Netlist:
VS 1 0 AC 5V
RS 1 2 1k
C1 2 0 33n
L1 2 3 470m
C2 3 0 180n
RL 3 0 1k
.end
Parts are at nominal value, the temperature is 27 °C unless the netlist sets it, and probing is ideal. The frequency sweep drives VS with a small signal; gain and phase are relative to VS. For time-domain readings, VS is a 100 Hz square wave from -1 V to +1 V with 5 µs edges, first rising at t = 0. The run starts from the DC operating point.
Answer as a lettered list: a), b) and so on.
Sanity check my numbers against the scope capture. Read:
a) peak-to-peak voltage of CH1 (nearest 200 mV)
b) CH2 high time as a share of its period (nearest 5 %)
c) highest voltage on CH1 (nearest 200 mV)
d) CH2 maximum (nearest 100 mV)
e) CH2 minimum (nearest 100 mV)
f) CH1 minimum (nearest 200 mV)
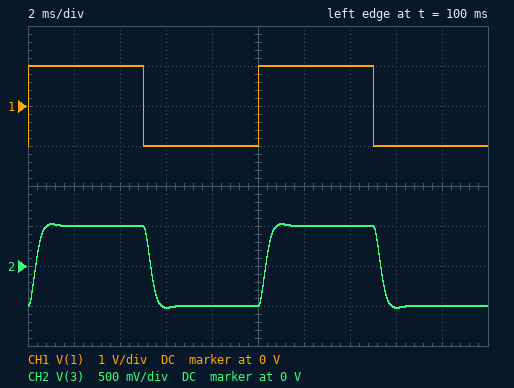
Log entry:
a) 2.0 V
b) 50 %
c) 1.0 V
d) 500 mV
e) -500 mV
f) -1.0 V
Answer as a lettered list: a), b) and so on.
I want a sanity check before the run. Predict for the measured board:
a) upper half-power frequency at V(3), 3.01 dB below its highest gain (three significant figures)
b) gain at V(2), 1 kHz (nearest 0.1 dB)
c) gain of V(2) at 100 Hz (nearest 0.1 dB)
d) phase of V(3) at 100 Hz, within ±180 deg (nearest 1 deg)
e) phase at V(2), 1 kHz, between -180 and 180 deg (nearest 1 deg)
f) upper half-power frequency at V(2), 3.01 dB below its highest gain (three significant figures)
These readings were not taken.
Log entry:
a) 719 Hz
b) -0.7 dB
c) -6.0 dB
d) -12 deg
e) 10 deg
f) 5.30 kHz
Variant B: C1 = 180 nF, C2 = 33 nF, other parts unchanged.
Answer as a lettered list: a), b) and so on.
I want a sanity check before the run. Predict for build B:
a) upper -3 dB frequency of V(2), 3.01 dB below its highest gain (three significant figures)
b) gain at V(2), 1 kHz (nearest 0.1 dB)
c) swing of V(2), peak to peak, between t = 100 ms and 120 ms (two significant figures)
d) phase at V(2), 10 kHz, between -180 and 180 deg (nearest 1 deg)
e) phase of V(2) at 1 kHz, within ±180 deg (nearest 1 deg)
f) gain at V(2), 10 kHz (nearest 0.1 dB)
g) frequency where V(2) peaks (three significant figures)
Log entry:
a) 1.49 kHz
b) -2.8 dB
c) 1.8 V
d) -85 deg
e) -36 deg
f) -21.1 dB
g) 707 Hz
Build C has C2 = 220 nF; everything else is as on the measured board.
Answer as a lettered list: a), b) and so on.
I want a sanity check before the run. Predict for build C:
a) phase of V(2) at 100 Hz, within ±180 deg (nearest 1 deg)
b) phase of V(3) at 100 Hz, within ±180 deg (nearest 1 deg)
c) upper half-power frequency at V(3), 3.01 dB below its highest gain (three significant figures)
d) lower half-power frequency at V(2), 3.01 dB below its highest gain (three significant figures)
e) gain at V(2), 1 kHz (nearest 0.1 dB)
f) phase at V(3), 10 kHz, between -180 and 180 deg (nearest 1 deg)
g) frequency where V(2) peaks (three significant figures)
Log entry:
a) 4 deg
b) -13 deg
c) 680 Hz
d) 577 Hz
e) -0.6 dB
f) 120 deg
g) 1.52 kHz
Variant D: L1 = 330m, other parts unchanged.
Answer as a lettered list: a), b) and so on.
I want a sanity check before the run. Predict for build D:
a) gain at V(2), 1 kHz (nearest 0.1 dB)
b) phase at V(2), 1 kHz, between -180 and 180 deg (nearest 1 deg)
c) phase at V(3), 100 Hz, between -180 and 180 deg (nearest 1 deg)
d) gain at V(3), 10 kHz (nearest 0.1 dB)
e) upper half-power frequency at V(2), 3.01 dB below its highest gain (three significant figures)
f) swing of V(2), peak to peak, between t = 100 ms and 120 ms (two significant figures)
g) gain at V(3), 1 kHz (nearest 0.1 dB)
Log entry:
a) -1.8 dB
b) 18 deg
c) -10 deg
d) -54.5 dB
e) 5.45 kHz
f) 2.4 V
g) -9.6 dB
